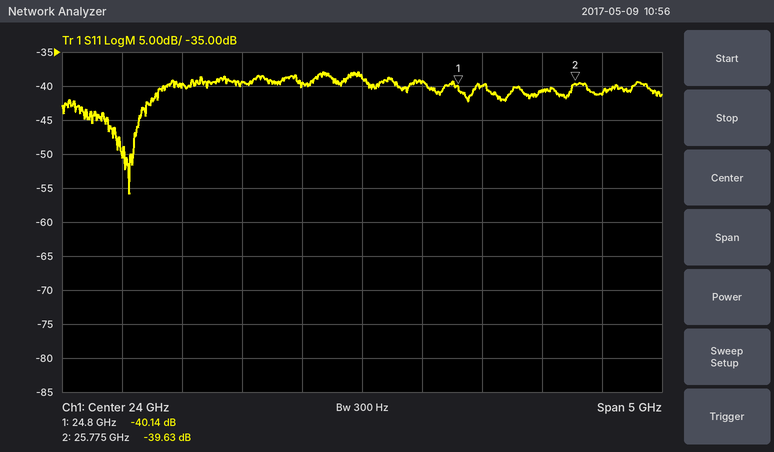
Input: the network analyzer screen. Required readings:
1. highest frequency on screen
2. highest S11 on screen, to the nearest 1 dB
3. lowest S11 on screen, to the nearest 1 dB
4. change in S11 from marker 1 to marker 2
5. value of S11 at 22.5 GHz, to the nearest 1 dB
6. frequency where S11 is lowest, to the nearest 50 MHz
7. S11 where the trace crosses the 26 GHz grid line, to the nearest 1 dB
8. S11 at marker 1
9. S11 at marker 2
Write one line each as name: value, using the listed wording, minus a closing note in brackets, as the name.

highest frequency on screen: 26.5 GHz
highest S11 on screen, to the nearest 1 dB: -38 dB
lowest S11 on screen, to the nearest 1 dB: -56 dB
change in S11 from marker 1 to marker 2: 0.51 dB
value of S11 at 22.5 GHz, to the nearest 1 dB: -40 dB
frequency where S11 is lowest, to the nearest 50 MHz: 22.05 GHz
S11 where the trace crosses the 26 GHz grid line, to the nearest 1 dB: -41 dB
S11 at marker 1: -40.14 dB
S11 at marker 2: -39.63 dB
